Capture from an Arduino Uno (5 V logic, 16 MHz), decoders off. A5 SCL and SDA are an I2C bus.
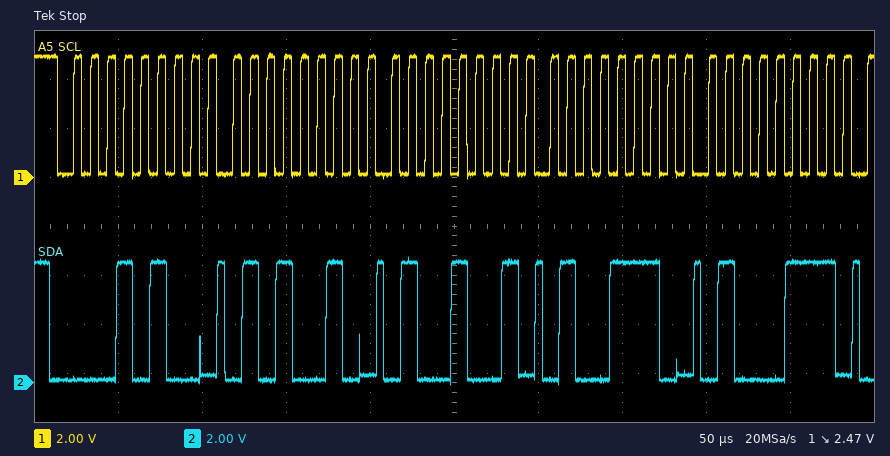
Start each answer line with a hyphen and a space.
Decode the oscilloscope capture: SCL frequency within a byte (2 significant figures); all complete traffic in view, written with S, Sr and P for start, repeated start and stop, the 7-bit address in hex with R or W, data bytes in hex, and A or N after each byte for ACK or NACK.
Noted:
- 100 kHz
- S 0AW A 52 A 49 A 4E A 47 A
